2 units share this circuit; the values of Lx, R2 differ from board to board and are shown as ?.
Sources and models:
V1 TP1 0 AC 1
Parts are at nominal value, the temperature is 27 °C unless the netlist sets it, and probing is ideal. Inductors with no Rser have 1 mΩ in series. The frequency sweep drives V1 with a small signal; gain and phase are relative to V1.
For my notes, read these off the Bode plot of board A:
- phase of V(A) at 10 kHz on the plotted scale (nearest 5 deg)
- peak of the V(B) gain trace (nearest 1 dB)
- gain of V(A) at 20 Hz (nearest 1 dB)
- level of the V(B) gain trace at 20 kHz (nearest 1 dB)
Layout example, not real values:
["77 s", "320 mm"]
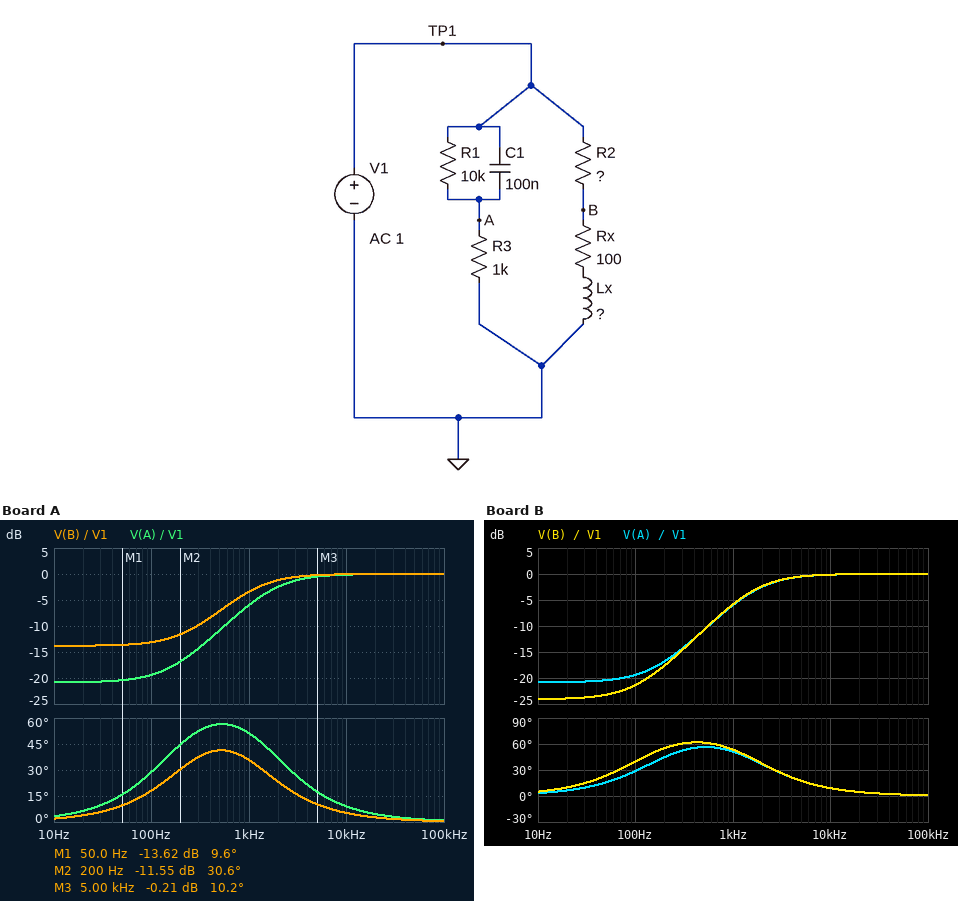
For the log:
["10 deg", "0 dB", "-21 dB", "0 dB"]
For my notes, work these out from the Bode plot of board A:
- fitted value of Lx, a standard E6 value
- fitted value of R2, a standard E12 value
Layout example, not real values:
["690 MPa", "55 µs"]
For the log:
["68 mH", "390 Ω"]
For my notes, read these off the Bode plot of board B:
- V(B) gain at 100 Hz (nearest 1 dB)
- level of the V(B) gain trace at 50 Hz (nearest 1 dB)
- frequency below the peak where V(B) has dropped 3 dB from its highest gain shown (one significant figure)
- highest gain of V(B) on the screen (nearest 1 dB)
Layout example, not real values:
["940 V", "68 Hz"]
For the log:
["-21 dB", "-23 dB", "2 kHz", "0 dB"]
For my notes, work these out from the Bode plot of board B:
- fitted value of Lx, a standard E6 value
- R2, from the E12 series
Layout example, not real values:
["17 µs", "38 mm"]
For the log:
["150 mH", "1.5 kΩ"]
